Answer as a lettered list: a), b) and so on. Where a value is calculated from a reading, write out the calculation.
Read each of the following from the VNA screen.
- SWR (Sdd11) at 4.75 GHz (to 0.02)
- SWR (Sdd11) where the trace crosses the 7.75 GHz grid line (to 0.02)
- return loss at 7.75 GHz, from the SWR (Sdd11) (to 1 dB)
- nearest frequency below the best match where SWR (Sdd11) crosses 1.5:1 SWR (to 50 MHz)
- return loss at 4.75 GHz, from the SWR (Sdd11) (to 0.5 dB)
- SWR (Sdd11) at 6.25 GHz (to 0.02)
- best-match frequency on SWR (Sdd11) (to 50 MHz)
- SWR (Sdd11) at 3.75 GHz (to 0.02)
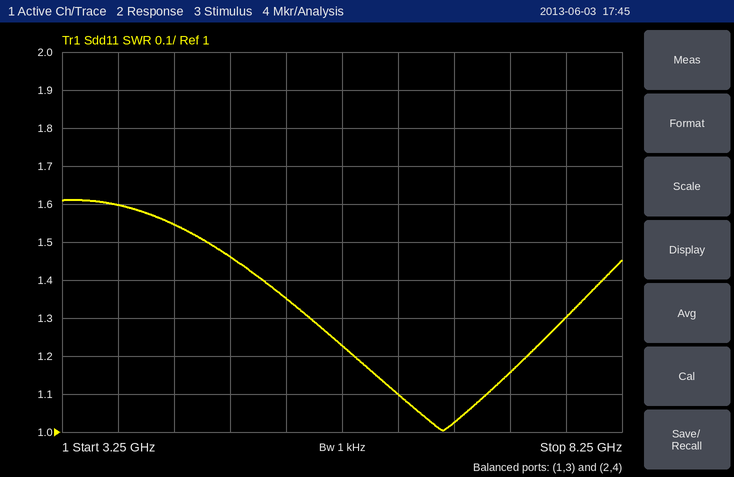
a) 1.46
b) 1.30
c) −20 log10((1.3 − 1)/(1.3 + 1)) ≈ 18 dB
d) 4.55 GHz
e) −20 log10((1.46 − 1)/(1.46 + 1)) ≈ 14.6 dB, so 14.5 dB to the nearest 0.5 dB
f) 1.10
g) 6.65 GHz
h) 1.60
